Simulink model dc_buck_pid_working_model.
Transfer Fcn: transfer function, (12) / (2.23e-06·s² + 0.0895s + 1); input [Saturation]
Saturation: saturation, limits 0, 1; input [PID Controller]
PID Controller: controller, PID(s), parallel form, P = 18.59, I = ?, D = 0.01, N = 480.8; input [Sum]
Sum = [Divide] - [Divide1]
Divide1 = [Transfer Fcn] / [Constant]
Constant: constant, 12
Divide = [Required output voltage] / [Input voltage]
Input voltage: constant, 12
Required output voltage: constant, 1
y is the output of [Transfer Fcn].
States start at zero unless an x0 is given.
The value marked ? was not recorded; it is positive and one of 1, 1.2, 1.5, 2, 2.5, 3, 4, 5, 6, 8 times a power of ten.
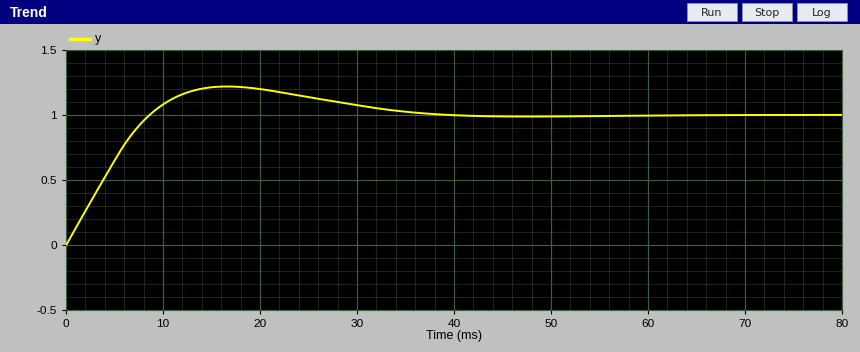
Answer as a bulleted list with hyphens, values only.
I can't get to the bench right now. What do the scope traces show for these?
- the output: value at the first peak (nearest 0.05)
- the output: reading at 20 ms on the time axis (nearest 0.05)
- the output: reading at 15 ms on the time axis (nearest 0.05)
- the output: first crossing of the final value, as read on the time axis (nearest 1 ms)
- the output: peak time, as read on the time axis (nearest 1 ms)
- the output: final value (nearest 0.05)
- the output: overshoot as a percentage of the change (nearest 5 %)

- 1.20
- 1.20
- 1.20
- 9 ms
- 17 ms
- 1.00
- 20 %
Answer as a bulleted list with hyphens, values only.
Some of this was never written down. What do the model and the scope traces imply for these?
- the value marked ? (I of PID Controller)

- 2000
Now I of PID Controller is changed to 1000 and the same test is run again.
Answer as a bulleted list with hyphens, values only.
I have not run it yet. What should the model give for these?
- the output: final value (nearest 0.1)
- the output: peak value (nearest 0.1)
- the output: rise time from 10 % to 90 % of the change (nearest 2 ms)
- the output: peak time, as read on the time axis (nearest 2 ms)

- 1.0
- 1.1
- 8 ms
- 22 ms
